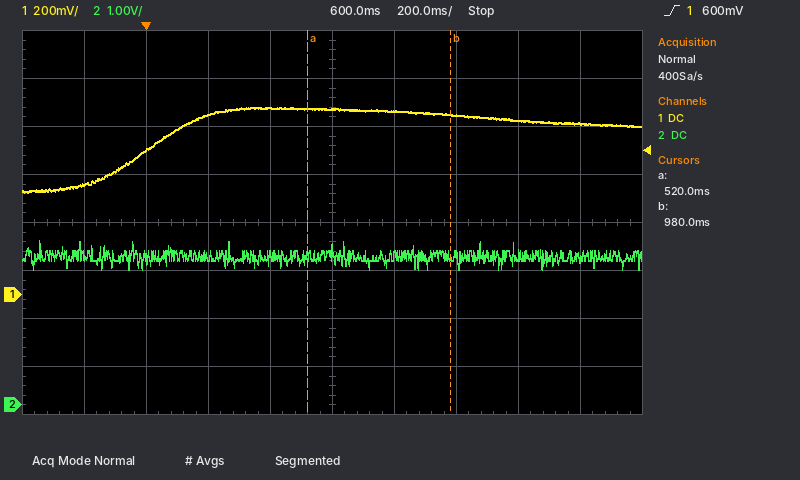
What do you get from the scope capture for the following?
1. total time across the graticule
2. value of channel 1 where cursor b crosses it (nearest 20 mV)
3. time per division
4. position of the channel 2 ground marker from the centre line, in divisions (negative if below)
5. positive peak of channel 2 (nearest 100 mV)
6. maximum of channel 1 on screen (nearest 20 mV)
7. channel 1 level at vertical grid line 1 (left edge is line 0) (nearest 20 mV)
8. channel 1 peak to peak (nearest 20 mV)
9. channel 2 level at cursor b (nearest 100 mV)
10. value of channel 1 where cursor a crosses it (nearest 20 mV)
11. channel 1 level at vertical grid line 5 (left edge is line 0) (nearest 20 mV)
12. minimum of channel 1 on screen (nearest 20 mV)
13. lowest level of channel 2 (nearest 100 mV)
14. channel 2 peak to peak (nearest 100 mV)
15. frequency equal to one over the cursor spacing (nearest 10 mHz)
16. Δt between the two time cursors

2 s
740 mV
200 ms
-3.8 div
3.4 V
780 mV
460 mV
360 mV
3.1 V
780 mV
780 mV
420 mV
2.8 V
600 mV
2.17 Hz
460 ms
